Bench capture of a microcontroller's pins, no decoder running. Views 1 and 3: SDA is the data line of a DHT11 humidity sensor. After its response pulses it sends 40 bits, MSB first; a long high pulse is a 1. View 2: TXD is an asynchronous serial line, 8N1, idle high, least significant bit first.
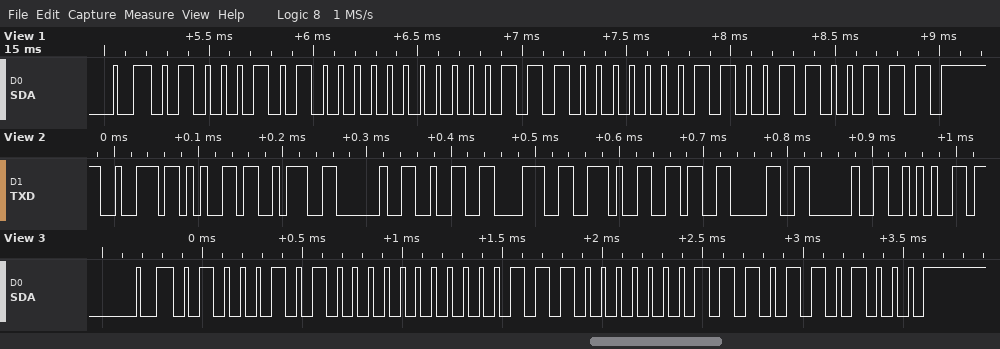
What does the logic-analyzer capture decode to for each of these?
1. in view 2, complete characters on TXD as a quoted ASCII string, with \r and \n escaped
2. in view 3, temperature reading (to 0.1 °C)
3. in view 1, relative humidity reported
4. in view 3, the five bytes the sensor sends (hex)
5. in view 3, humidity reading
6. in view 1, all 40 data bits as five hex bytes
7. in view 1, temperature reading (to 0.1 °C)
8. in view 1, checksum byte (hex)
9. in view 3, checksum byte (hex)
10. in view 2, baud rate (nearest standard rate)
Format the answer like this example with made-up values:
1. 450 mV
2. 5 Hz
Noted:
1. "re: 28.60 *"
2. 28.7 °C
3. 69 %
4. 45 00 1C 07 68
5. 69 %
6. 45 00 1C 06 67
7. 28.6 °C
8. 0x67
9. 0x68
10. 115200 baud
